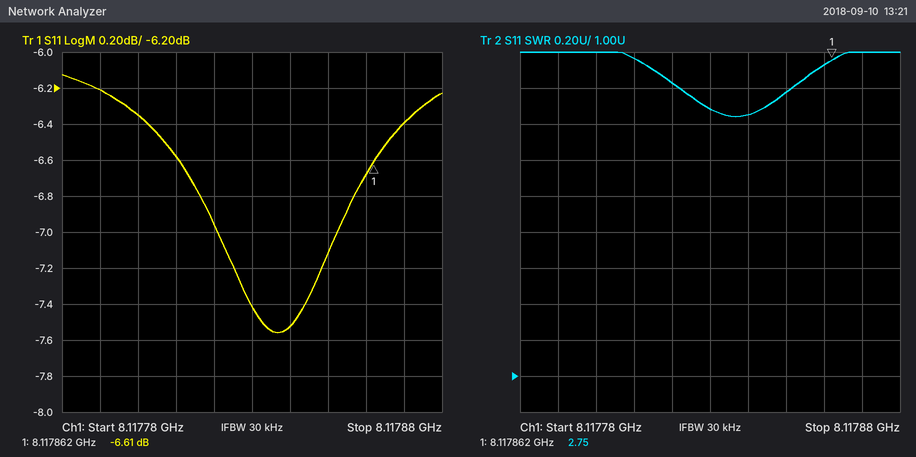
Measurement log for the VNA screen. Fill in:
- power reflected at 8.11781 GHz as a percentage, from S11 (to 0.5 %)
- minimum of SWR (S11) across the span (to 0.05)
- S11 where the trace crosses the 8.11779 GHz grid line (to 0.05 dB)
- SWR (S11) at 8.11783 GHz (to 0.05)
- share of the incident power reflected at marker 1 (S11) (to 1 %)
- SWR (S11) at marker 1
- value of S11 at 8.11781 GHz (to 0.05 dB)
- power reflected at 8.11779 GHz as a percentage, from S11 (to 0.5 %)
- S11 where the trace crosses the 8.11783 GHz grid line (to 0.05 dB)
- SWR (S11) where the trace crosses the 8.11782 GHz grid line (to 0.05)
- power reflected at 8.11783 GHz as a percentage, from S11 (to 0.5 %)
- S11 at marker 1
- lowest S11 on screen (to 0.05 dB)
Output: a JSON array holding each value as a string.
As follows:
["22.0 %", "2.45", "-6.20 dB", "2.50", "22 %", "2.75", "-6.60 dB", "24.0 %", "-7.40 dB", "2.65", "18.0 %", "-6.61 dB", "-7.55 dB"]
